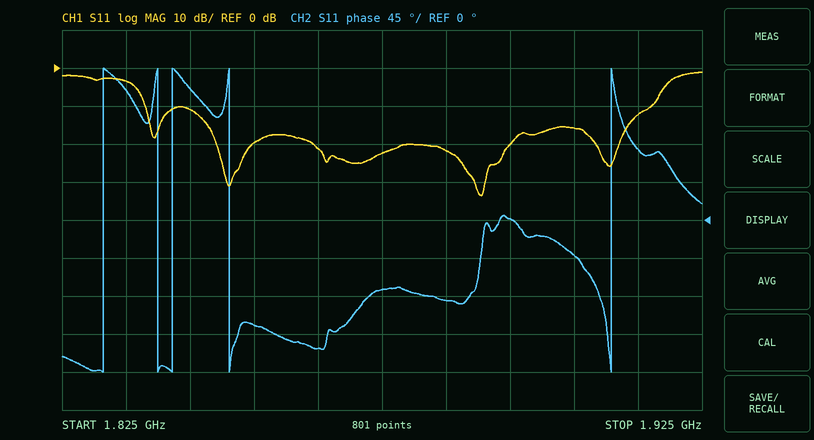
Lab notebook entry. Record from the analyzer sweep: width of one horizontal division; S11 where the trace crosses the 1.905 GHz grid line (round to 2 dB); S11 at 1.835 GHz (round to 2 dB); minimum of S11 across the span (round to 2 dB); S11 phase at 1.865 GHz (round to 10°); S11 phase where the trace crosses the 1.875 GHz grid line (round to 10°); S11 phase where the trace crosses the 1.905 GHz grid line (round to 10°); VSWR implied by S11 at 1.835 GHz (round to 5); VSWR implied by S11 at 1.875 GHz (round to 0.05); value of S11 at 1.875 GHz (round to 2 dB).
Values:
10 MHz
-16 dB
-4 dB
-34 dB
-150°
-80°
-40°
5
1.15
-22 dB
